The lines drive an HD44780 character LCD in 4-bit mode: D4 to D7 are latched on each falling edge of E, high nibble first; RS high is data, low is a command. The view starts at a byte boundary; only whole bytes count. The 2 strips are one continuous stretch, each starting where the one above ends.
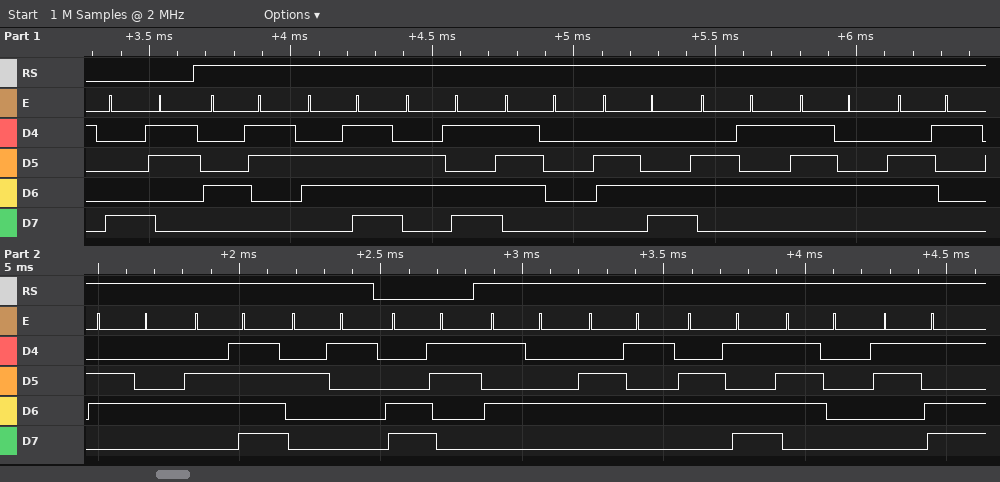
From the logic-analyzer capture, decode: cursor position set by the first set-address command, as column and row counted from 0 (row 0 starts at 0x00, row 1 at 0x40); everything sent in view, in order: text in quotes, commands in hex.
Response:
column 3, row 0
0x83 "Completado!" 0xC3 "Temp="
